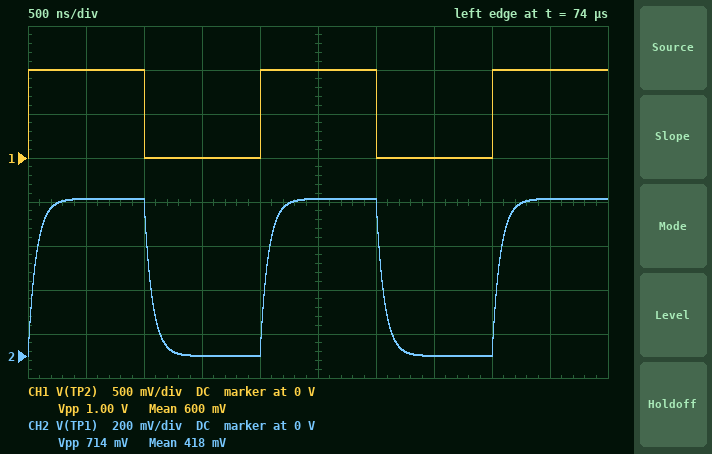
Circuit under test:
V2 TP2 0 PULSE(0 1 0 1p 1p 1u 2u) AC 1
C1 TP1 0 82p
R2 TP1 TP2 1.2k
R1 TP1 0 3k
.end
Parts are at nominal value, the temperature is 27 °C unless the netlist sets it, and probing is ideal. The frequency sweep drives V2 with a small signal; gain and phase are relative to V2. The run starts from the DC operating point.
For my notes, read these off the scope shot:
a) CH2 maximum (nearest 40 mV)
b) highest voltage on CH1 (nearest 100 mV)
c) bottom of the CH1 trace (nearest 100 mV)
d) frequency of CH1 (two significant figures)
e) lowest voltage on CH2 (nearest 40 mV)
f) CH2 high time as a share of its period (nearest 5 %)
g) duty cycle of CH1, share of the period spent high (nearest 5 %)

720 mV
1.0 V
0 V
500 kHz
0 V
50 %
50 %
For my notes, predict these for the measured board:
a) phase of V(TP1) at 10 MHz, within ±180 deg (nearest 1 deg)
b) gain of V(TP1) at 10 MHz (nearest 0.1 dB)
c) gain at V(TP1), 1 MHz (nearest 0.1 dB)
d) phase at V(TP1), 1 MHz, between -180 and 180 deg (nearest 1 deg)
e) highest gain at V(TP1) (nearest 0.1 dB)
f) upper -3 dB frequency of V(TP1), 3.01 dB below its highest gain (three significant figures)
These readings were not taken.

-77 deg
-16.0 dB
-3.7 dB
-24 deg
-2.9 dB
2.26 MHz
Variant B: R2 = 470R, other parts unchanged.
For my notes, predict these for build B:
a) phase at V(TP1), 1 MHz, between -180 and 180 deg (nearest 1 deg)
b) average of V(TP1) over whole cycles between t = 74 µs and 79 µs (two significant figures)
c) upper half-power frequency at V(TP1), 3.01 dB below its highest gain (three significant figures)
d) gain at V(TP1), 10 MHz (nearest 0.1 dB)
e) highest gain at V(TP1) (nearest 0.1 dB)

-12 deg
430 mV
4.78 MHz
-8.6 dB
-1.3 dB
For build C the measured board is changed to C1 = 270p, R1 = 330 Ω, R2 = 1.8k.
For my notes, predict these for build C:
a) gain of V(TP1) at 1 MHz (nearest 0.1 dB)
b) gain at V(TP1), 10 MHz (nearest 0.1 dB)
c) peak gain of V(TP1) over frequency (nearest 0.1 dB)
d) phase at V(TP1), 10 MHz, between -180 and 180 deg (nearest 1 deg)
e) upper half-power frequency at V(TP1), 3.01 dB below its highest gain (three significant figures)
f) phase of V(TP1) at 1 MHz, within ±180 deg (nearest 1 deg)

-17.1 dB
-29.9 dB
-16.2 dB
-78 deg
2.11 MHz
-25 deg
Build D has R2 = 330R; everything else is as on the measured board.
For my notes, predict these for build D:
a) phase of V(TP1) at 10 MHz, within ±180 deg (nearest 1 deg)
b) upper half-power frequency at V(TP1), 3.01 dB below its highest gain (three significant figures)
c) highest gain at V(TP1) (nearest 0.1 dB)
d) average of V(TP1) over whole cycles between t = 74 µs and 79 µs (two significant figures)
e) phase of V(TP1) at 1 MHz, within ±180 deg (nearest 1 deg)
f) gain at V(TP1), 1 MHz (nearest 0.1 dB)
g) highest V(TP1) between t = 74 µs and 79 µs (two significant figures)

-57 deg
6.53 MHz
-0.9 dB
450 mV
-9 deg
-1.0 dB
900 mV
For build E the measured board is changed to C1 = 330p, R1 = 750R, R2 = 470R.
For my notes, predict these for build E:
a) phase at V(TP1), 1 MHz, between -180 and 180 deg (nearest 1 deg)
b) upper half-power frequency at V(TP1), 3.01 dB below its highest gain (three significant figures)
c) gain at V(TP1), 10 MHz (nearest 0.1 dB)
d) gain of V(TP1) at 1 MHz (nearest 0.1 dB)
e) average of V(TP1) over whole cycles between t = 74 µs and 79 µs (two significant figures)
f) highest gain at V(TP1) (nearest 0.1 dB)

-31 deg
1.67 MHz
-19.9 dB
-5.6 dB
310 mV
-4.2 dB
